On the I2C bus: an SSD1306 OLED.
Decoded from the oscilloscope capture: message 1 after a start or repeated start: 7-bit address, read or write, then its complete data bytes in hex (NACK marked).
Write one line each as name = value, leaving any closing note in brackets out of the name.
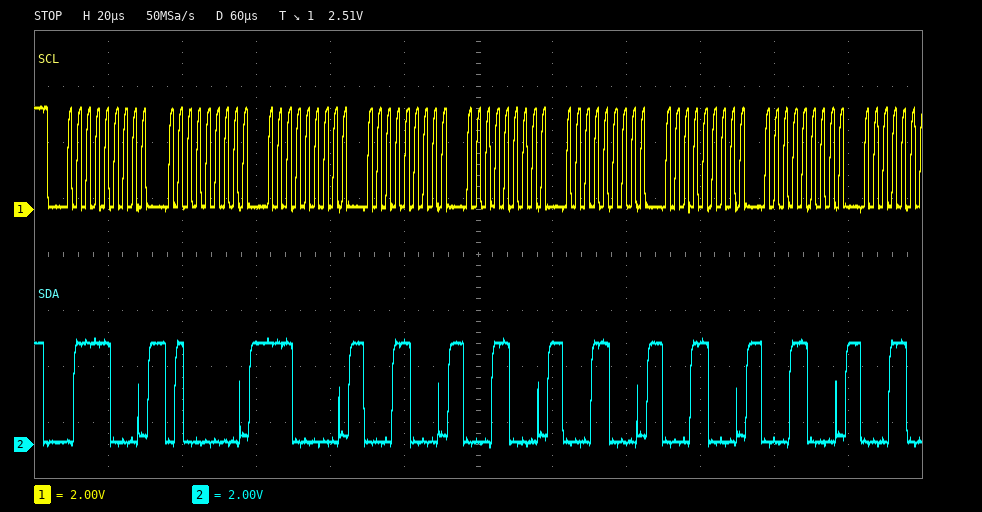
message 1 after a start or repeated start: 7-bit address, read or write, then its complete data bytes in hex = 0x3C write: 40 E0 18 18 18 18 18
